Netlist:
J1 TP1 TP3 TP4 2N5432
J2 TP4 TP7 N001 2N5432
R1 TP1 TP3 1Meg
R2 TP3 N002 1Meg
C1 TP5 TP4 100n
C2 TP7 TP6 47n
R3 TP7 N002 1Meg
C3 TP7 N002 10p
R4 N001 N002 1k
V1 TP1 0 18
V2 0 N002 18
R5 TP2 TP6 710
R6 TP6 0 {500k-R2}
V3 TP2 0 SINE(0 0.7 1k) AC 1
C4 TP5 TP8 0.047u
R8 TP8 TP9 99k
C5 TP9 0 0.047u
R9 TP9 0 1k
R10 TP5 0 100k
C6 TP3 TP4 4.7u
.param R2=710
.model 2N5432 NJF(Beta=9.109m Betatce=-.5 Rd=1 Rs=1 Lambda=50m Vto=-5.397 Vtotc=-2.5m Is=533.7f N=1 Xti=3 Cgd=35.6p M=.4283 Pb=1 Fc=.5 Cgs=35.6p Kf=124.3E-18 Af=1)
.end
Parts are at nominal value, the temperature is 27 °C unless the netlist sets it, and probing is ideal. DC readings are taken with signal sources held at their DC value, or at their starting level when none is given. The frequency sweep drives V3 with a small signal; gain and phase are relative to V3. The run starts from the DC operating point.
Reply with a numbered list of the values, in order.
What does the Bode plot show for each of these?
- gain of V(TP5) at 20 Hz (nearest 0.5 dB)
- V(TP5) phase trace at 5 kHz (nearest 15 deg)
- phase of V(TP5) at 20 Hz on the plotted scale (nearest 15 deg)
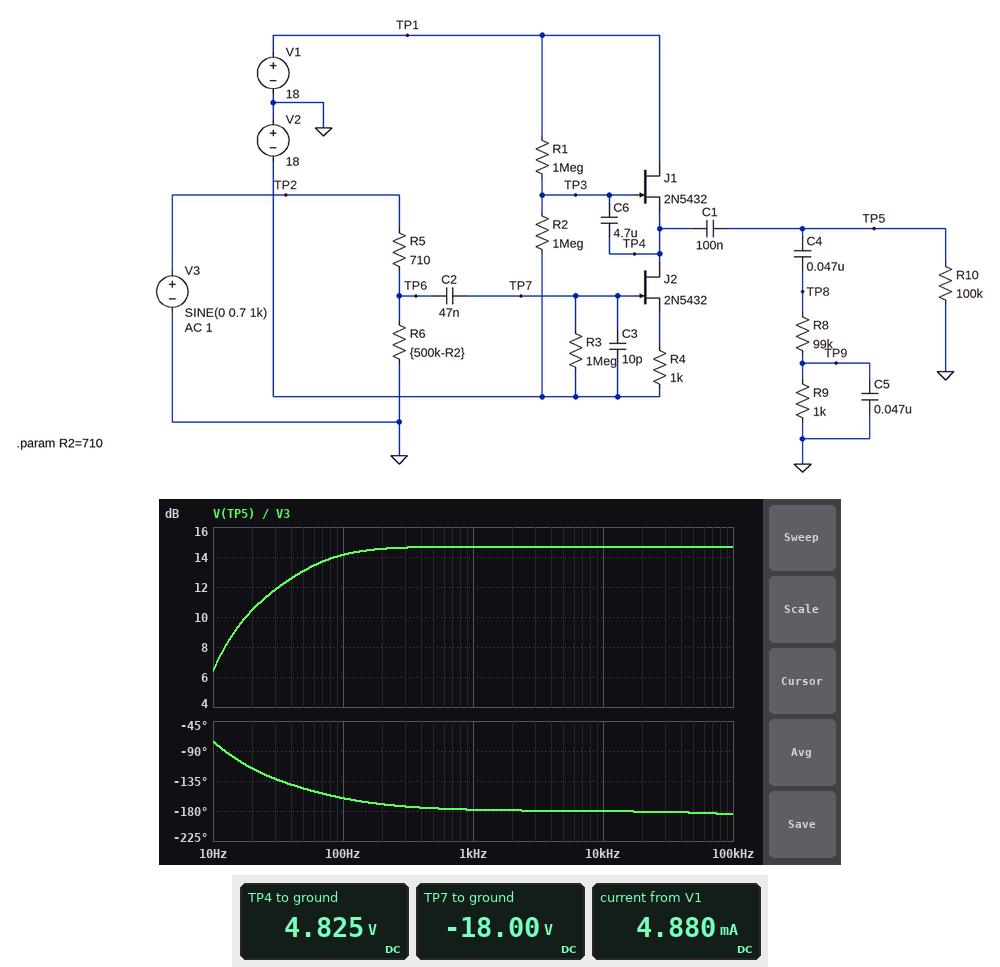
1. 10.5 dB
2. -180 deg
3. -120 deg
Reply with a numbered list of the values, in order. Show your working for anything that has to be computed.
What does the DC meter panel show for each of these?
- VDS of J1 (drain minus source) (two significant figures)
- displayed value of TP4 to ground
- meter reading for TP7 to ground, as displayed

1. 18 V - 4.825 V = 13 V
2. 4.825 V
3. -18.00 V
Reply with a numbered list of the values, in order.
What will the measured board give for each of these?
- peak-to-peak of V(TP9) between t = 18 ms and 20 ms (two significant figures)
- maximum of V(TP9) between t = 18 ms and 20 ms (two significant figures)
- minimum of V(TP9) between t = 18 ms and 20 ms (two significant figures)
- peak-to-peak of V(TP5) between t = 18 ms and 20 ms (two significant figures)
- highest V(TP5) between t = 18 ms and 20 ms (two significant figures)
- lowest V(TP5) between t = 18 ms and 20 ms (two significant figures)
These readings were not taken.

1. 73 mV
2. 36 mV
3. -36 mV
4. 7.6 V
5. 3.8 V
6. -3.8 V
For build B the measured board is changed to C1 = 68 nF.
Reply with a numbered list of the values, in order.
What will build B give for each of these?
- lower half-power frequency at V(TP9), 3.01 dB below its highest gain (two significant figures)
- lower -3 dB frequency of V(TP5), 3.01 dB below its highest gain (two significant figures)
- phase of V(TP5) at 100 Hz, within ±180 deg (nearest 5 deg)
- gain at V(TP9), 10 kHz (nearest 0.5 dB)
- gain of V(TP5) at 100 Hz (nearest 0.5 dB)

1. 62 Hz
2. 45 Hz
3. -155 deg
4. -35.0 dB
5. 13.5 dB
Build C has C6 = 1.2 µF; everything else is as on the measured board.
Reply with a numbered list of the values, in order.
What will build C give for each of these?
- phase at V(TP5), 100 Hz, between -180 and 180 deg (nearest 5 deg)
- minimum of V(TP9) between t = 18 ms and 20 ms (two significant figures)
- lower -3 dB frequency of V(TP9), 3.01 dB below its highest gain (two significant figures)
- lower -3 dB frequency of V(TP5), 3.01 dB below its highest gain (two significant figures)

1. -150 deg
2. -36 mV
3. 59 Hz
4. 45 Hz
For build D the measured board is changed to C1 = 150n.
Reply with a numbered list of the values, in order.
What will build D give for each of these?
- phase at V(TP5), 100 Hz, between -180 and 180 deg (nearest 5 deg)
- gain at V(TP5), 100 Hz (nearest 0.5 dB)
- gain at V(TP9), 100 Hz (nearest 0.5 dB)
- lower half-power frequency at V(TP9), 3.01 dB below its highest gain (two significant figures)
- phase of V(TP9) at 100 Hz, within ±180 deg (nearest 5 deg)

1. -165 deg
2. 14.5 dB
3. -26.0 dB
4. 44 Hz
5. -150 deg
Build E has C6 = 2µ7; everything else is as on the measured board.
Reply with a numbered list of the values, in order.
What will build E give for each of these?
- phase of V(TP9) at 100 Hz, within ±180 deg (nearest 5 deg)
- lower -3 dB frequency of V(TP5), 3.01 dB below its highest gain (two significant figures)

1. -140 deg
2. 32 Hz
